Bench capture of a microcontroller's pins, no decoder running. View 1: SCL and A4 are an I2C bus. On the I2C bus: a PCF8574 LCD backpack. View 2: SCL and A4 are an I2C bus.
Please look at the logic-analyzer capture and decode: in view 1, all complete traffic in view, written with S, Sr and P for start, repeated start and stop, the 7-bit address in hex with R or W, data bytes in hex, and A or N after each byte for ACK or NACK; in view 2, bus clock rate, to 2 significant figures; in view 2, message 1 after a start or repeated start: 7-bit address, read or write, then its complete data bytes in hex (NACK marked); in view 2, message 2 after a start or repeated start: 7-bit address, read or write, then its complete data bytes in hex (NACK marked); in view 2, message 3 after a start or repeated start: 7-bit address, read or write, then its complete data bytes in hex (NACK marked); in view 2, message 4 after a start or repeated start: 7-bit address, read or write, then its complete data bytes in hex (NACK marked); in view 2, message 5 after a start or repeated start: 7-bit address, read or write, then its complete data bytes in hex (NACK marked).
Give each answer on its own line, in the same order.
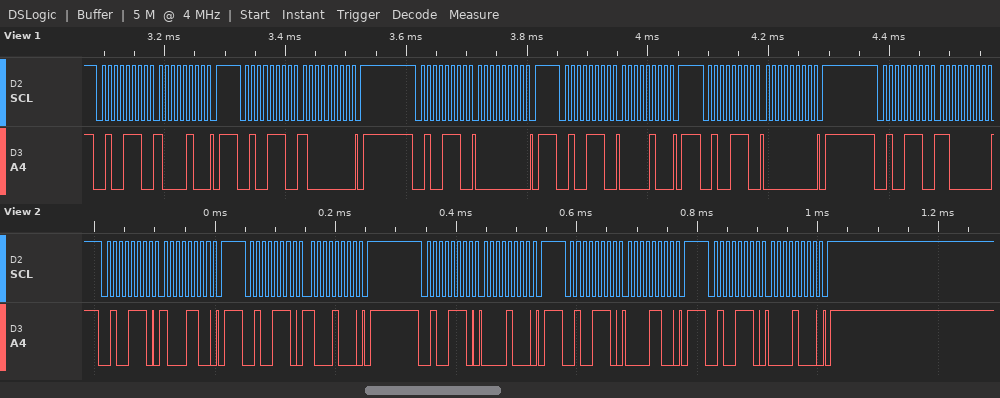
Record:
S 27W A 84 A P S 27W A 80 A P S 27W A 00 A P S 27W A 04 A P S 27W A 00 A P S 27W A C0 A
100 kHz
0x27 write: 8C
0x27 write: 88
0x27 write: 08
0x27 write: 0C
0x27 write: 08
